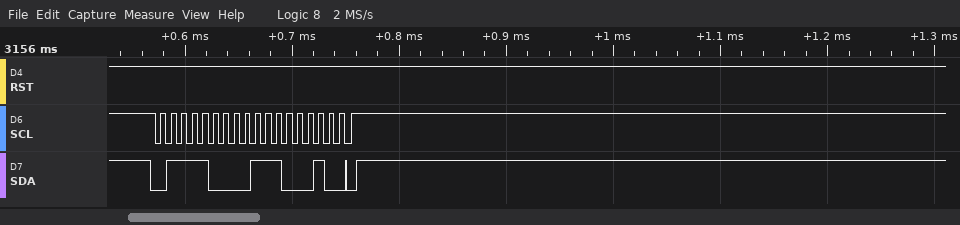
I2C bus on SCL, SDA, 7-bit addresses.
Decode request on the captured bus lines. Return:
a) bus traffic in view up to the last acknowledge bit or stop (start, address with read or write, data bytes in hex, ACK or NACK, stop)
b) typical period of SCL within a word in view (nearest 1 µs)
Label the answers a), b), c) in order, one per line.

a) start, address 3C write ACK, E2 ACK, stop
b) 10 µs
